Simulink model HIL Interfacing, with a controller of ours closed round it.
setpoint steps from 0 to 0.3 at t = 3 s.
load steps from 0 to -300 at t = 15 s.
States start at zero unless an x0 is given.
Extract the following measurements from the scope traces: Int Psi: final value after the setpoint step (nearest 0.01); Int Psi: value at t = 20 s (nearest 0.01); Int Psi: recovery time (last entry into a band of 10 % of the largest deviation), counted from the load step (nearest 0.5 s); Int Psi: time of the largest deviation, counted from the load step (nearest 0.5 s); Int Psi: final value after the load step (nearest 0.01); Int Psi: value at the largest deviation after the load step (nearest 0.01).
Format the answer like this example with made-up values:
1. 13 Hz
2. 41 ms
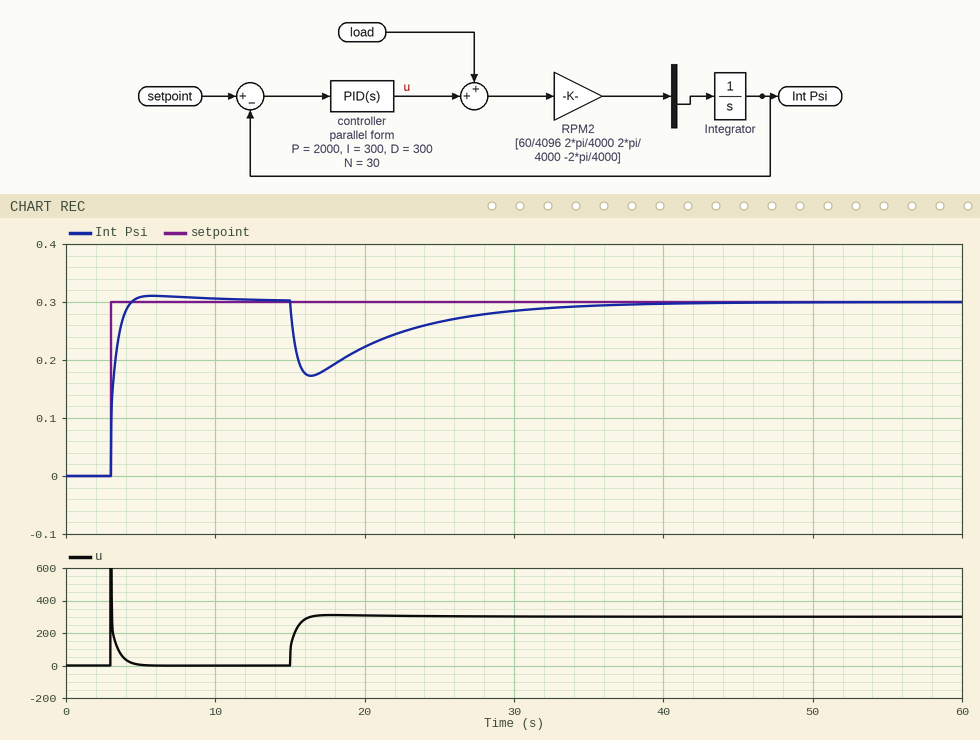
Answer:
1. 0.30
2. 0.22
3. 16.0 s
4. 1.5 s
5. 0.30
6. 0.17
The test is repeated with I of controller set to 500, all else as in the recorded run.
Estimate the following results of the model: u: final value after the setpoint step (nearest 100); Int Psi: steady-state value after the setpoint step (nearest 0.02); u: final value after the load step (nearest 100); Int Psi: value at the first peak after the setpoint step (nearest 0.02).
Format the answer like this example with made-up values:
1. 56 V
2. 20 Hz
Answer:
1. 0
2. 0.30
3. 300
4. 0.32
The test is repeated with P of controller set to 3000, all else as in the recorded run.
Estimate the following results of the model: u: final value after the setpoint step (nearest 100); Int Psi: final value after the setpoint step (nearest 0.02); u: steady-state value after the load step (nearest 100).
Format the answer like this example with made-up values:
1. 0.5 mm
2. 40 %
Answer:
1. 0
2. 0.30
3. 300
